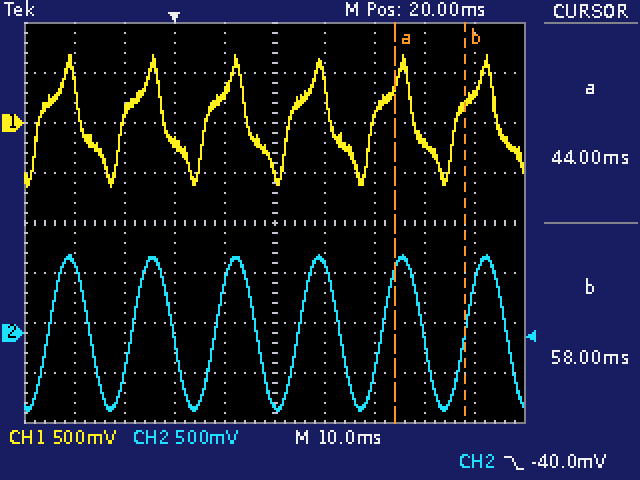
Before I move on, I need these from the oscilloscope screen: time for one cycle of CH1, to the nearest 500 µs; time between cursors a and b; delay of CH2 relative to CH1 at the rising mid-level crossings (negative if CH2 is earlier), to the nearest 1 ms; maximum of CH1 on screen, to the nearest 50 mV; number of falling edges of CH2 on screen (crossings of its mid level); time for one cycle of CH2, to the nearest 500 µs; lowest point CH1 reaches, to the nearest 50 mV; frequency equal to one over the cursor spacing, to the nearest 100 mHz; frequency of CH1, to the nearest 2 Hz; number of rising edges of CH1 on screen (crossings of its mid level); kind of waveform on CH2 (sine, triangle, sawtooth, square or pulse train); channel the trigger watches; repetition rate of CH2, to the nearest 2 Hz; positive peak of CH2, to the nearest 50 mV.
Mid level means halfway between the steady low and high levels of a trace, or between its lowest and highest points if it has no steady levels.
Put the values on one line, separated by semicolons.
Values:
16.5 ms; 14 ms; +2 ms; 700 mV; 6; 16.5 ms; -650 mV; 71.4 Hz; 60 Hz; 6; sine; CH2; 60 Hz; 800 mV
